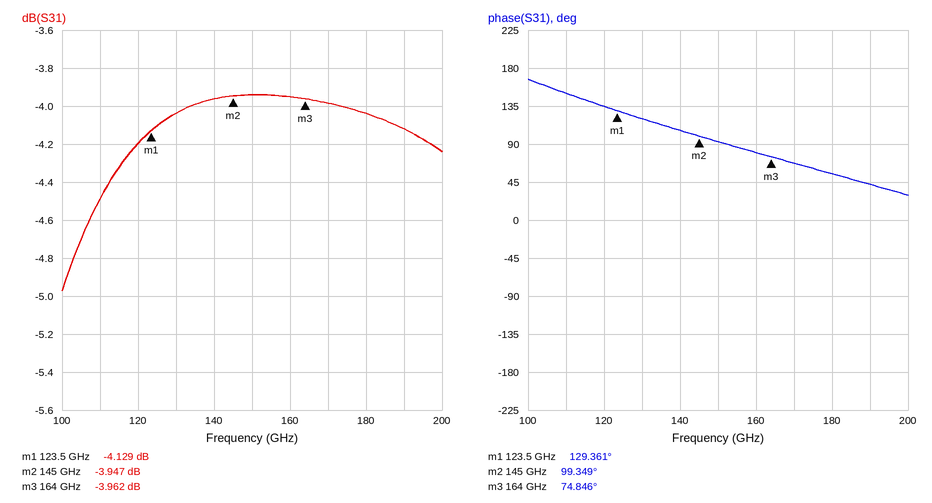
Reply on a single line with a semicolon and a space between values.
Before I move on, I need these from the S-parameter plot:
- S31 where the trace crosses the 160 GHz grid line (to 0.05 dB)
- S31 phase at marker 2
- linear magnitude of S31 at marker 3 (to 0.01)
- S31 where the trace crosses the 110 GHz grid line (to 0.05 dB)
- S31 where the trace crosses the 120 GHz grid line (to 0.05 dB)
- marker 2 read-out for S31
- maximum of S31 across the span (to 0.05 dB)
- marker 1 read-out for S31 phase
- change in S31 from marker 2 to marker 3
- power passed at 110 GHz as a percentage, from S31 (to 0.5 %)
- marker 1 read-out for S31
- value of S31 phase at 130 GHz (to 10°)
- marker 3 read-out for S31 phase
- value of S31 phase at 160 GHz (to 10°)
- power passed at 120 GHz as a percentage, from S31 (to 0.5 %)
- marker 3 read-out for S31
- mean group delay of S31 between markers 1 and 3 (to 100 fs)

-3.95 dB; 99.349°; 0.63; -4.50 dB; -4.20 dB; -3.947 dB; -3.95 dB; 129.361°; -0.015 dB; 35.5 %; -4.129 dB; 120°; 74.846°; 80°; 38.0 %; -3.962 dB; 3.7 ps
